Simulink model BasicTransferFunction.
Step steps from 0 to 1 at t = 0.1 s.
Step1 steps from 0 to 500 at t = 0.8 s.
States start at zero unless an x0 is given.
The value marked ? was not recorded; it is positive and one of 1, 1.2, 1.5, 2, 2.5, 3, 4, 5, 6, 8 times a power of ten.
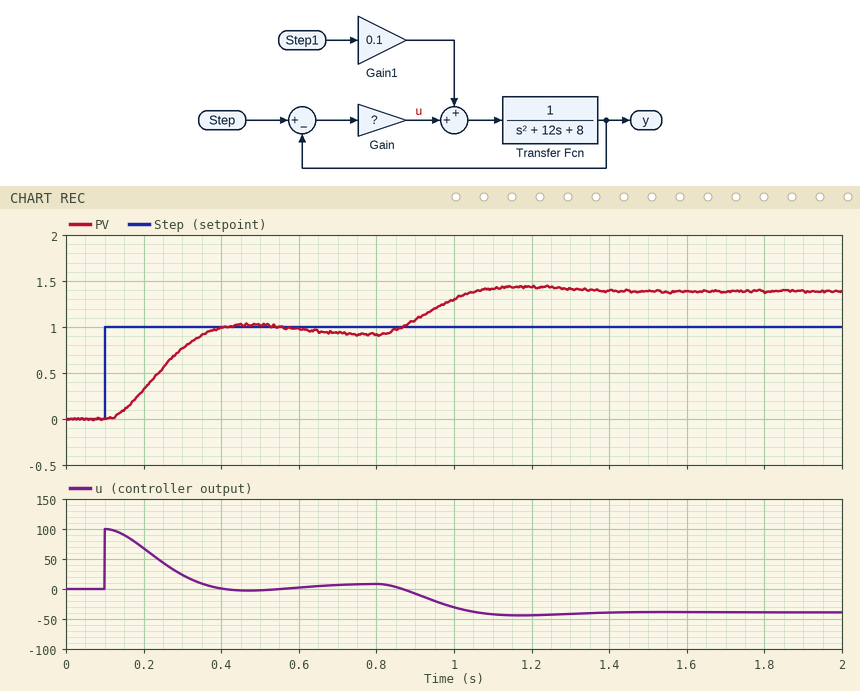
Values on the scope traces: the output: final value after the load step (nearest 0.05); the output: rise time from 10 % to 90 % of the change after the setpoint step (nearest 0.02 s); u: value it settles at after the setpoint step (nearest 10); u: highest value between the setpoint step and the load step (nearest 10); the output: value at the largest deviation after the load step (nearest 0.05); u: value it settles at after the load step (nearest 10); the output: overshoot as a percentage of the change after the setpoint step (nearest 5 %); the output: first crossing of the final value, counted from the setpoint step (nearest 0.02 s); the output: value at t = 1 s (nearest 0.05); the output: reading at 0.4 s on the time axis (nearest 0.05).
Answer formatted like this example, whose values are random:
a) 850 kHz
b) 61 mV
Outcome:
a) 1.40
b) 0.18 s
c) 10
d) 100
e) 1.45
f) -40
g) 10 %
h) 0.26 s
i) 1.30
j) 1.00
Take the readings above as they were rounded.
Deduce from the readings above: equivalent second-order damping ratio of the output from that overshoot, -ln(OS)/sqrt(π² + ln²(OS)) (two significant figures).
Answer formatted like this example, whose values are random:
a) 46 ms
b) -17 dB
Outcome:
a) 0.59
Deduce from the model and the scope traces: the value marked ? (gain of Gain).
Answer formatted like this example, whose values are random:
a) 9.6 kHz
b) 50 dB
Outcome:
a) 100
